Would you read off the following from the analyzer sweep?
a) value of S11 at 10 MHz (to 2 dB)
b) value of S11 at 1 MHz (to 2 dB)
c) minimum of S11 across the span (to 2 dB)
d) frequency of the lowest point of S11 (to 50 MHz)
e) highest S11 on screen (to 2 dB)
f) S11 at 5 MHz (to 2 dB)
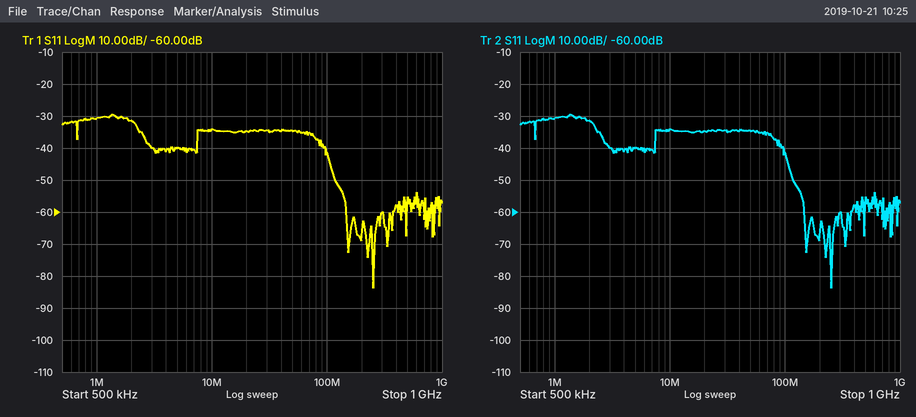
-34 dB
-30 dB
-84 dB
250 MHz
-30 dB
-40 dB
